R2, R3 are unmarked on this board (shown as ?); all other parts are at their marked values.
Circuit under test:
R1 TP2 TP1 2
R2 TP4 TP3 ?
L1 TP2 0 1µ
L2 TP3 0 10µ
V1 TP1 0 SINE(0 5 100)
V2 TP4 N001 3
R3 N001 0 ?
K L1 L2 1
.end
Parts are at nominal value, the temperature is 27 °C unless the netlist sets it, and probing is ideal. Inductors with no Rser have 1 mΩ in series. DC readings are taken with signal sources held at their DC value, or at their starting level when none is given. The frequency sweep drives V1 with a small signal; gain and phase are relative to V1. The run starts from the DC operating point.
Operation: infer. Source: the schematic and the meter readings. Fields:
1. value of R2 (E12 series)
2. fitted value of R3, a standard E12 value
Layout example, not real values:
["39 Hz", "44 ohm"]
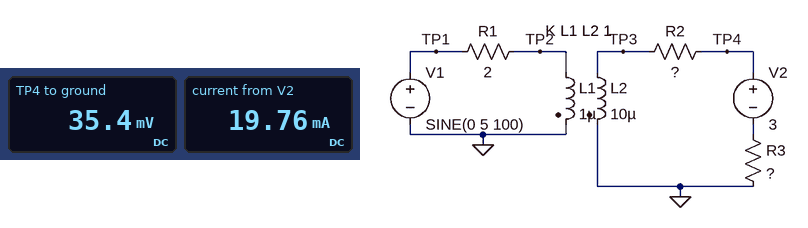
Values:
["1.8 Ω", "150 Ω"]
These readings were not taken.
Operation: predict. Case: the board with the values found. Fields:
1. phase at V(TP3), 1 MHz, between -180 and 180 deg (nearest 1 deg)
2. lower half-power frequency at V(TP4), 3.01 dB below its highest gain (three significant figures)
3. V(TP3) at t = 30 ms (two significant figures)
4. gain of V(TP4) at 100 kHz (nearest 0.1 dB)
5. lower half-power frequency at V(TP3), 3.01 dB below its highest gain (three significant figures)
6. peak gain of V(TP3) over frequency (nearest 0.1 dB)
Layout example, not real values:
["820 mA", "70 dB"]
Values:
["16 deg", "281 kHz", "5.0 mV", "-0.7 dB", "281 kHz", "8.9 dB"]
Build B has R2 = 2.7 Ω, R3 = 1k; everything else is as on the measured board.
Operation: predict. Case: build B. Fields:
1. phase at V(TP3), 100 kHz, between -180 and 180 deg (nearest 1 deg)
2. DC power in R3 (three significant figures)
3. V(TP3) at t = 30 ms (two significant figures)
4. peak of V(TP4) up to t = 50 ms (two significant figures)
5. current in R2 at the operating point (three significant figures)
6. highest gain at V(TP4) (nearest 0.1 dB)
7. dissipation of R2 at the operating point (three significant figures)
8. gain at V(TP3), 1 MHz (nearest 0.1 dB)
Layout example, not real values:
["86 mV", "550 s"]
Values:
["72 deg", "8.95 mW", "5.0 mV", "13 mV", "2.99 mA", "9.8 dB", "24.2 µW", "9.4 dB"]
